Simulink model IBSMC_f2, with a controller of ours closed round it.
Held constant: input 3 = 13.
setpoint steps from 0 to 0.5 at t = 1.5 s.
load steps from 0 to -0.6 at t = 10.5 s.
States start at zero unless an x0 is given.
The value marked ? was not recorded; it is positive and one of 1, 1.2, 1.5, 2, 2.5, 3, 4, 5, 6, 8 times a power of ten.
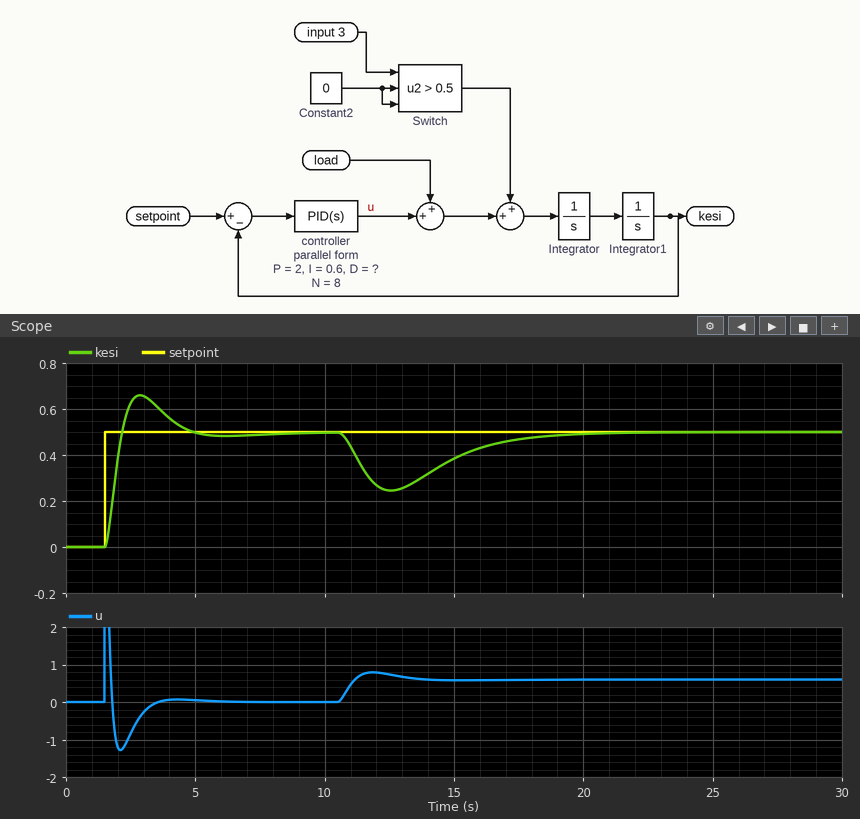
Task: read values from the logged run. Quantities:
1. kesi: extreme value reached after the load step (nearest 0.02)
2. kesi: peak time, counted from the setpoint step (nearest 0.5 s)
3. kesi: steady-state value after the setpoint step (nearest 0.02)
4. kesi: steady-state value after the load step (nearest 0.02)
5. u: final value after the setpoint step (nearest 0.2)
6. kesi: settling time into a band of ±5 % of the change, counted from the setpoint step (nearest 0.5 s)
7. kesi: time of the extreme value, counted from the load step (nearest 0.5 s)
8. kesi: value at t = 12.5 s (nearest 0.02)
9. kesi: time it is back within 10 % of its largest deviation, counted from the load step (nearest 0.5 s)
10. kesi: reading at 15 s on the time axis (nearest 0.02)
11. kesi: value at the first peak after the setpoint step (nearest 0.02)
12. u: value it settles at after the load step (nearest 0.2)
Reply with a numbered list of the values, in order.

1. 0.24
2. 1.5 s
3. 0.50
4. 0.50
5. 0.0
6. 3.0 s
7. 2.0 s
8. 0.24
9. 7.5 s
10. 0.38
11. 0.66
12. 0.6
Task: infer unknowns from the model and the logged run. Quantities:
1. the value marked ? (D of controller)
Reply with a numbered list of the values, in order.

1. 2
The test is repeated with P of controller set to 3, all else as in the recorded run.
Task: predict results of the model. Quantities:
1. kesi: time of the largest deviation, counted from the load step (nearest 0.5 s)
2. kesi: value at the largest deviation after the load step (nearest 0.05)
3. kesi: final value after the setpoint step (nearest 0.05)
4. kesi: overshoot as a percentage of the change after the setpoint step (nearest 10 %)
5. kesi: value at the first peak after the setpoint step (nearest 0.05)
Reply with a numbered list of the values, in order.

1. 1.5 s
2. 0.30
3. 0.50
4. 40 %
5. 0.70
